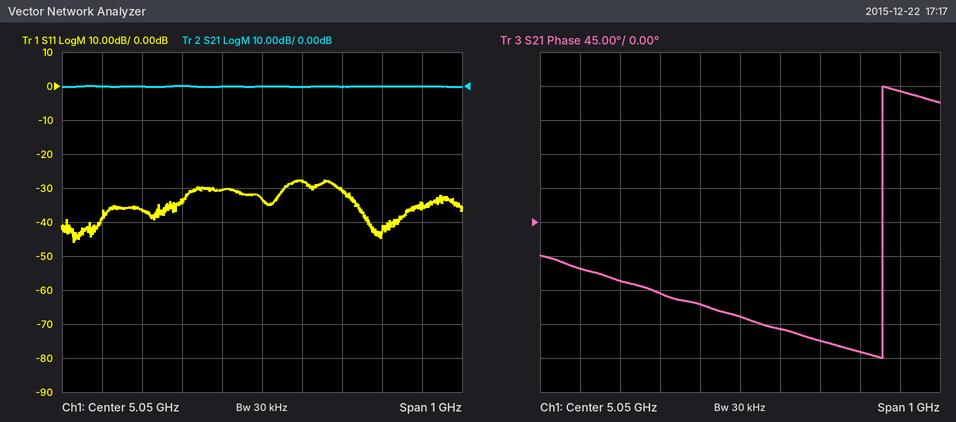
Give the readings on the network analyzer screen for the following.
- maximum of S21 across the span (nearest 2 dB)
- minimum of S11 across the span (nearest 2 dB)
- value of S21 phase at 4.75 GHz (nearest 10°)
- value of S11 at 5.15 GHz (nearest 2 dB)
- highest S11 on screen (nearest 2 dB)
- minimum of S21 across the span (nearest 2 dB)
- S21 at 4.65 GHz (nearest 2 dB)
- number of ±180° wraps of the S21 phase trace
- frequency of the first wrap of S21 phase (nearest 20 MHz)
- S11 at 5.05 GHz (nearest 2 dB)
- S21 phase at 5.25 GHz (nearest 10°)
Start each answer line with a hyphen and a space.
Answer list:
- 0 dB
- -46 dB
- -80°
- -28 dB
- -28 dB
- 0 dB
- 0 dB
- 1
- 5.40 GHz
- -34 dB
- -160°
